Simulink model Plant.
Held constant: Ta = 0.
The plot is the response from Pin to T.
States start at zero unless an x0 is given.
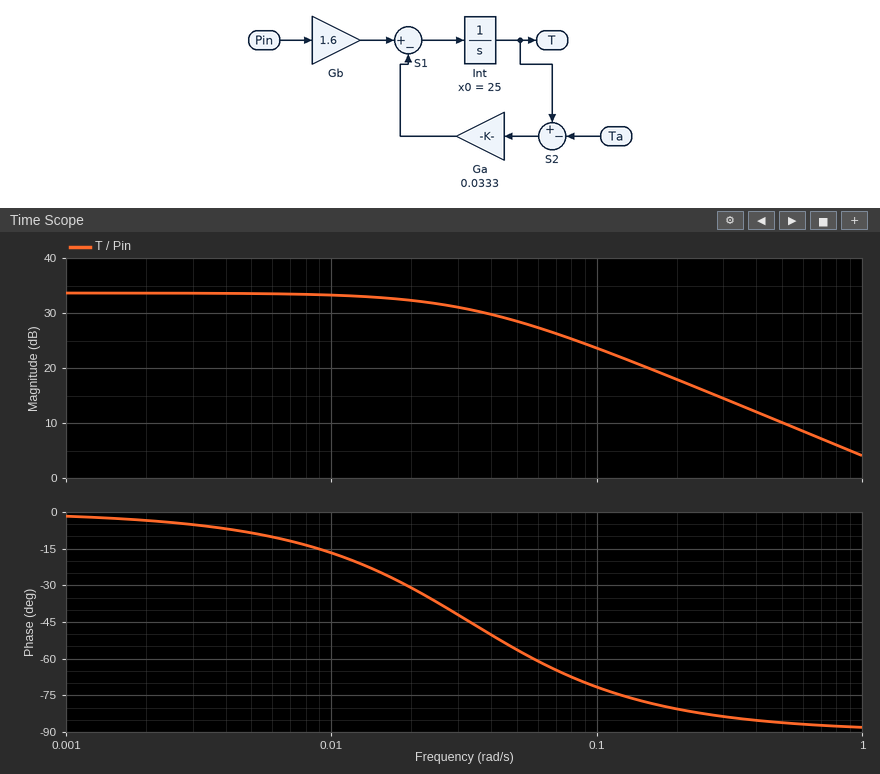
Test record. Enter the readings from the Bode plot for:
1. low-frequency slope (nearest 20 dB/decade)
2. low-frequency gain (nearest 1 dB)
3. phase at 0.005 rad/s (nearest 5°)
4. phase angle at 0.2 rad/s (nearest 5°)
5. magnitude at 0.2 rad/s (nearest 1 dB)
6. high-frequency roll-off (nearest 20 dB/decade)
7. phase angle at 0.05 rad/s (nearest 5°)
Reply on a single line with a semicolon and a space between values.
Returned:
0 dB/decade; 34 dB; -10°; -80°; 18 dB; -20 dB/decade; -55°
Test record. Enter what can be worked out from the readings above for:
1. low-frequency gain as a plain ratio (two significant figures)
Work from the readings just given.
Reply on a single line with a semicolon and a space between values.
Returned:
50
